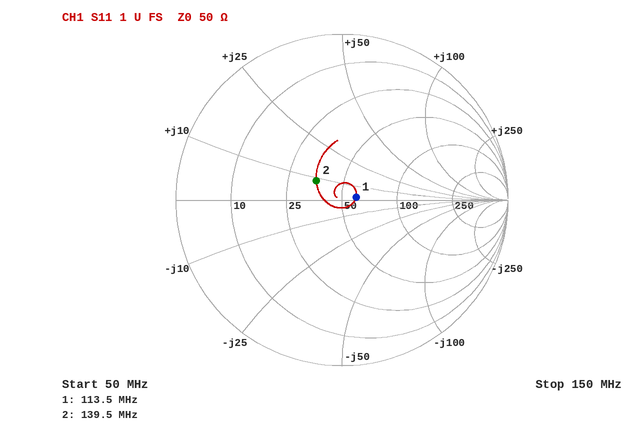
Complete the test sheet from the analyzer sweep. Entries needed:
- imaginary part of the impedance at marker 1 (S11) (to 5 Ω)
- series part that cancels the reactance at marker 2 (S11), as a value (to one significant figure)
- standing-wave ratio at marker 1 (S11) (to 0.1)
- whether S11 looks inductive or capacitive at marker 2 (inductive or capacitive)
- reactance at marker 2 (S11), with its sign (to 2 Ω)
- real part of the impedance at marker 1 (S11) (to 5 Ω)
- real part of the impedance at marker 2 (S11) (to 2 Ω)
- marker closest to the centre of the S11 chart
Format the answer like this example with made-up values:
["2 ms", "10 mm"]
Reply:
["0 Ω", "100 pF", "1.2", "inductive", "+8 Ω", "60 Ω", "36 Ω", "marker 1"]
